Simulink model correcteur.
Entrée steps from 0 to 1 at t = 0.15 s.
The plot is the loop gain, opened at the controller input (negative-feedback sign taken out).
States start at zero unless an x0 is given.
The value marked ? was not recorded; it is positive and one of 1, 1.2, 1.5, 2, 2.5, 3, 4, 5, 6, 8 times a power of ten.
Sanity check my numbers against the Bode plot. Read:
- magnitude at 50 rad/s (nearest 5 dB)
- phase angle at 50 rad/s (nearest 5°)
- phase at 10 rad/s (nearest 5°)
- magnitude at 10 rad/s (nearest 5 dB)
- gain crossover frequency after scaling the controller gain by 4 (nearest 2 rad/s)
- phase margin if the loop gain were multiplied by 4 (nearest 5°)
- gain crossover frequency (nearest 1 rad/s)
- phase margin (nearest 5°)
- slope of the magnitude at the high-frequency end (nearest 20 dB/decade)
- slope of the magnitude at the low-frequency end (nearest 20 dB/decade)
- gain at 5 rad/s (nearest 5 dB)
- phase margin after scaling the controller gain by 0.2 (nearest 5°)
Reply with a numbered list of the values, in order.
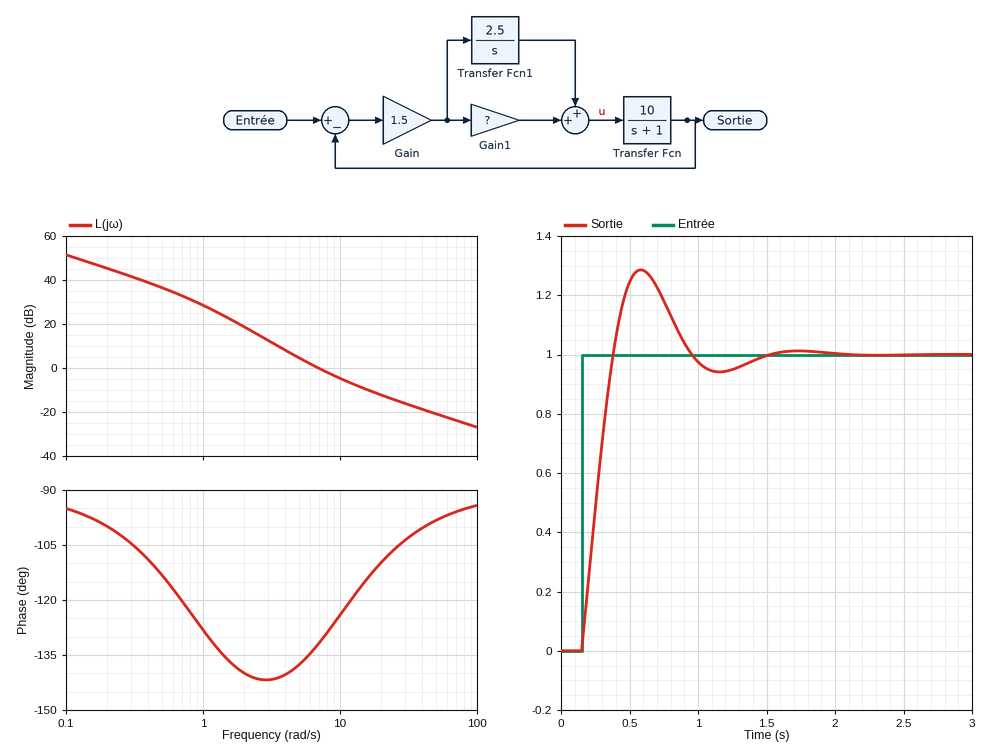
1. -20 dB
2. -100°
3. -125°
4. -5 dB
5. 20 rad/s
6. 70°
7. 7 rad/s
8. 50°
9. -20 dB/decade
10. -20 dB/decade
11. 5 dB
12. 40°
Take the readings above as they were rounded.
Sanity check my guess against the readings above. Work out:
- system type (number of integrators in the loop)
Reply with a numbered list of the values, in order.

1. 1
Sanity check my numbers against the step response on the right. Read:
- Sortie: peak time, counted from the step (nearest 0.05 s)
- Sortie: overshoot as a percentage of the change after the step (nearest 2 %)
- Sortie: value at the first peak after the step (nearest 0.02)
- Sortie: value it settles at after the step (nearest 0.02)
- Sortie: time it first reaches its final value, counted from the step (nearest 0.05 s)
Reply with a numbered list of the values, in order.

1. 0.45 s
2. 28 %
3. 1.28
4. 1.00
5. 0.25 s
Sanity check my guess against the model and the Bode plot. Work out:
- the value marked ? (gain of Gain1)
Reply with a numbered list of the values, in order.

1. 0.3
